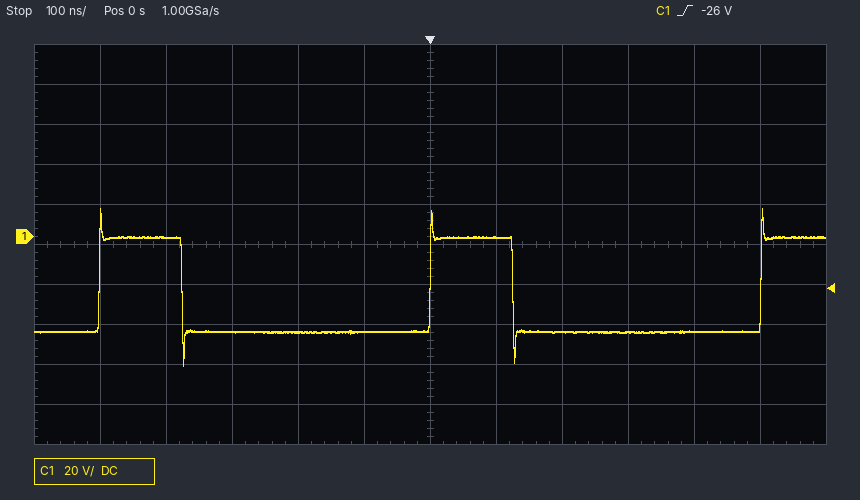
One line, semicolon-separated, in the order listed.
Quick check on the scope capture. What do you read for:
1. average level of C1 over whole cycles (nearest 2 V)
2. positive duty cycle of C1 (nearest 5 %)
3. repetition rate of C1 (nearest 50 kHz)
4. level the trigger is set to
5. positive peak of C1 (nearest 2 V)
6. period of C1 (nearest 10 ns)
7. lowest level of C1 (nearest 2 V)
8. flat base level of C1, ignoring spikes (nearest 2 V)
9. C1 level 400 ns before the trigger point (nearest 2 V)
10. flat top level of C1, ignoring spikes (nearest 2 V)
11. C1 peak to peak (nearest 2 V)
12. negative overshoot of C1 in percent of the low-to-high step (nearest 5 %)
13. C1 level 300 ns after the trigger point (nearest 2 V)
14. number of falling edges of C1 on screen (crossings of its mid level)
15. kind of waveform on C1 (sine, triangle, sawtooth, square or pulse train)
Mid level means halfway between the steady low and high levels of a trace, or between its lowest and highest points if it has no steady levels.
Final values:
-36 V; 25 %; 2.00 MHz; -26 V; 14 V; 500 ns; -64 V; -48 V; 0 V; 0 V; 78 V; 35 %; -48 V; 2; pulse train
